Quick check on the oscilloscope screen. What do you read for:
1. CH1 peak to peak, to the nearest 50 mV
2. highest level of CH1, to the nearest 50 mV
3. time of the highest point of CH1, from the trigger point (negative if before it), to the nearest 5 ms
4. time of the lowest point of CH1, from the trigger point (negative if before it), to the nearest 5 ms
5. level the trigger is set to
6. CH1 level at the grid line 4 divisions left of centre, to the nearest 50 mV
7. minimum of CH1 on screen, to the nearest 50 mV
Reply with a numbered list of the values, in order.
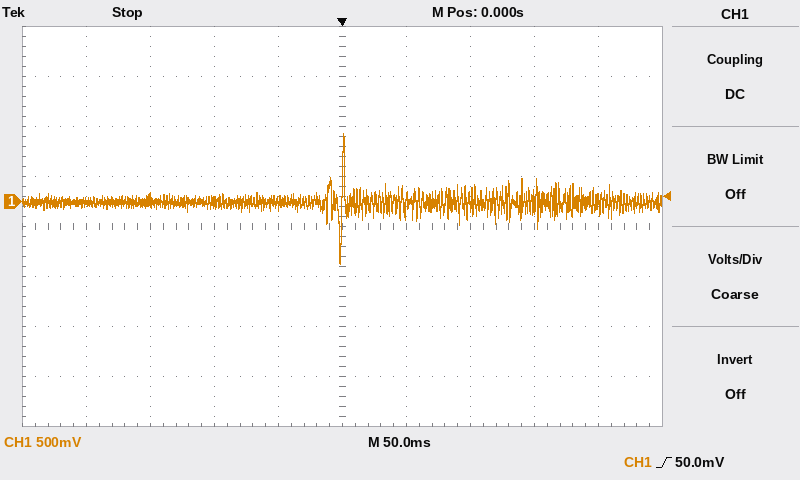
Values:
1. 1.30 V
2. 700 mV
3. 0 ms
4. 0 ms
5. 50.0 mV
6. 0 mV
7. -600 mV
